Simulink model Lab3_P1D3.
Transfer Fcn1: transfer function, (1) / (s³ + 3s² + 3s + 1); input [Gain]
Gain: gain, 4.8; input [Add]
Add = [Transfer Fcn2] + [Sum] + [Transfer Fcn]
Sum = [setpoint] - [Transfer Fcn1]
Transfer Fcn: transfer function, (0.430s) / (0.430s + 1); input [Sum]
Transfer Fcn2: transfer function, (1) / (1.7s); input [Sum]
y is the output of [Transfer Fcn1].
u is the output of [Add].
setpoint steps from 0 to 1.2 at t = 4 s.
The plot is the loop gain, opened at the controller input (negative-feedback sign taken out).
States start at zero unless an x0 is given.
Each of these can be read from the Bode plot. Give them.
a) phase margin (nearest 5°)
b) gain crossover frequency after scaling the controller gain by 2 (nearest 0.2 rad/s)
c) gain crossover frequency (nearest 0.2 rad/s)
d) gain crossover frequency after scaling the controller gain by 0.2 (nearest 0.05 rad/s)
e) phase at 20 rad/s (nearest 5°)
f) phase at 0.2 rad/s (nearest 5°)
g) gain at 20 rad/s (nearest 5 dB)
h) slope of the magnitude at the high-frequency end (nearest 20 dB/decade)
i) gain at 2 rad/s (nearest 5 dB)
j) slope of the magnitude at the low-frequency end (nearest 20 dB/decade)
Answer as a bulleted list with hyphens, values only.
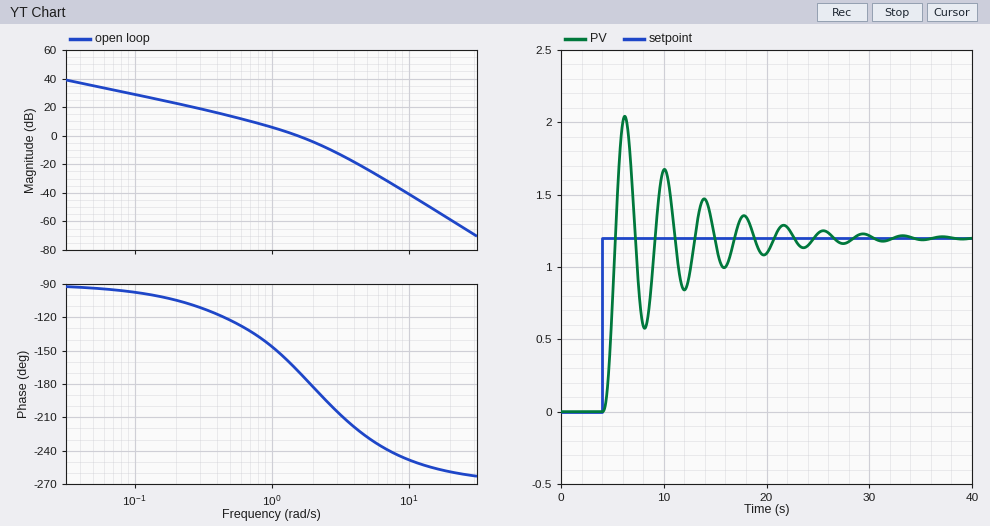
- 10°
- 2.2 rad/s
- 1.6 rad/s
- 0.50 rad/s
- -260°
- -105°
- -60 dB
- -60 dB/decade
- -5 dB
- -20 dB/decade
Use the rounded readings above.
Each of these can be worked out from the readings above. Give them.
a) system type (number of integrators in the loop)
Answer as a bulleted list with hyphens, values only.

- 1
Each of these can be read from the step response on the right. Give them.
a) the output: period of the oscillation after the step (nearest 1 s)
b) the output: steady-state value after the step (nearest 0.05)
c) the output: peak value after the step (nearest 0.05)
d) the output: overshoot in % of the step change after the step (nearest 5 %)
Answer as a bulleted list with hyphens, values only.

- 4 s
- 1.20
- 2.05
- 70 %
